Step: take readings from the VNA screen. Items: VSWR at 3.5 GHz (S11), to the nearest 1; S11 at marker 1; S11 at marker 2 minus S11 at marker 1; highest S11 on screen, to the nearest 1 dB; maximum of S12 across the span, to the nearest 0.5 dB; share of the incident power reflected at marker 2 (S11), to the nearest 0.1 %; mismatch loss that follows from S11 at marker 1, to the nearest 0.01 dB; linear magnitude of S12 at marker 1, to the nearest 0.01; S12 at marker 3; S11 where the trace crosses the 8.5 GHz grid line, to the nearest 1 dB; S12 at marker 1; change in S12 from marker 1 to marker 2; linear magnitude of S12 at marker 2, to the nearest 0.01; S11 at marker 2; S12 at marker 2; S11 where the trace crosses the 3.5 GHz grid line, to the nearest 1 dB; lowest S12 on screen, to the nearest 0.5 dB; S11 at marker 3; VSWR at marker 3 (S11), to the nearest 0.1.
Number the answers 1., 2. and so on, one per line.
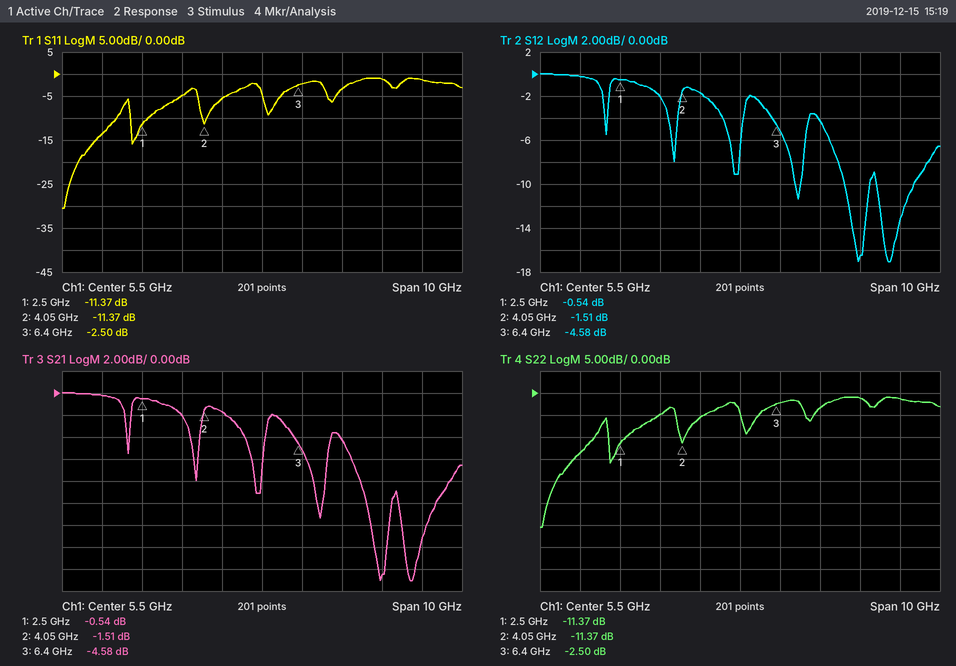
1. 4
2. -11.37 dB
3. 0.00 dB
4. -1 dB
5. 0.0 dB
6. 7.3 %
7. 0.33 dB
8. 0.94
9. -4.58 dB
10. -1 dB
11. -0.54 dB
12. -0.97 dB
13. 0.84
14. -11.37 dB
15. -1.51 dB
16. -5 dB
17. -17.0 dB
18. -2.50 dB
19. 7.0
